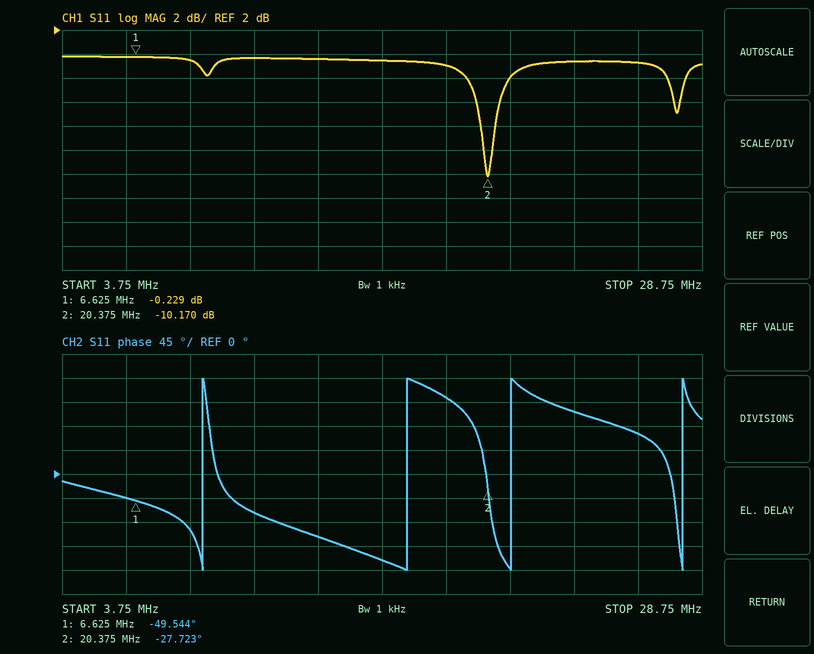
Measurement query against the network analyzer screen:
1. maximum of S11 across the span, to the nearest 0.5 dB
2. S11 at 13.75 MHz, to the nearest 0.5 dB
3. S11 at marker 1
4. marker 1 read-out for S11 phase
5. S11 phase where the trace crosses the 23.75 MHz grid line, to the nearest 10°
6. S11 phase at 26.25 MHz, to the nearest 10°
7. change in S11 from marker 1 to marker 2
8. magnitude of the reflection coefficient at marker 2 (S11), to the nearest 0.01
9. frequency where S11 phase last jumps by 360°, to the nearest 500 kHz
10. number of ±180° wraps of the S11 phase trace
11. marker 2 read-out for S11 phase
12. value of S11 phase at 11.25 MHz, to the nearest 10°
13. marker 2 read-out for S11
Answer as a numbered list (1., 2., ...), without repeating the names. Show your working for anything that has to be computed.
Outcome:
1. 0.0 dB
2. -0.5 dB
3. -0.229 dB
4. -49.544°
5. 120°
6. 80°
7. -10.17 − (-0.229) = -9.941 dB
8. 10^(-10.17/20) ≈ 0.31
9. 28.0 MHz
10. 4
11. -27.723°
12. -70°
13. -10.170 dB
